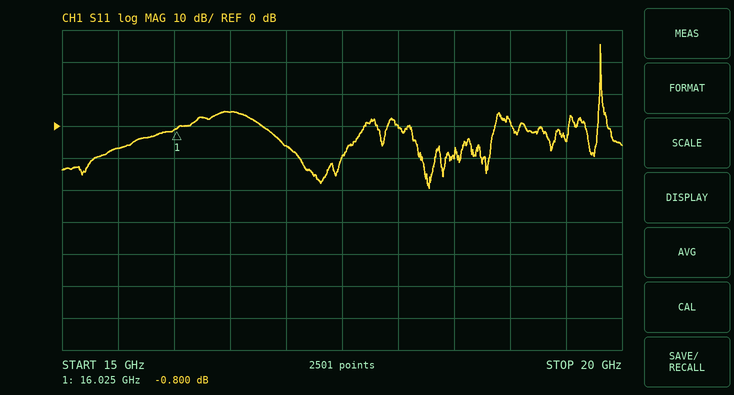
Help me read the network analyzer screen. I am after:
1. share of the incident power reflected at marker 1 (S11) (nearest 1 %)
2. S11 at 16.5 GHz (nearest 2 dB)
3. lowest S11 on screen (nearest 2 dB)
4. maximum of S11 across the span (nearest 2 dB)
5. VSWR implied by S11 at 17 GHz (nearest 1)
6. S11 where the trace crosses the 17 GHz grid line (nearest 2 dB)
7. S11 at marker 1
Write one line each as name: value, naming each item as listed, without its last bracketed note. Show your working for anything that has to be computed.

share of the incident power reflected at marker 1 (S11): 10^(-0.8/10) ≈ 83 %
S11 at 16.5 GHz: 4 dB
lowest S11 on screen: -20 dB
maximum of S11 across the span: 26 dB
VSWR implied by S11 at 17 GHz: |Γ| = 10^(-6/20) = 0.5012; VSWR = (1 + 0.5012)/(1 − 0.5012) ≈ 3
S11 where the trace crosses the 17 GHz grid line: -6 dB
S11 at marker 1: -0.800 dB
